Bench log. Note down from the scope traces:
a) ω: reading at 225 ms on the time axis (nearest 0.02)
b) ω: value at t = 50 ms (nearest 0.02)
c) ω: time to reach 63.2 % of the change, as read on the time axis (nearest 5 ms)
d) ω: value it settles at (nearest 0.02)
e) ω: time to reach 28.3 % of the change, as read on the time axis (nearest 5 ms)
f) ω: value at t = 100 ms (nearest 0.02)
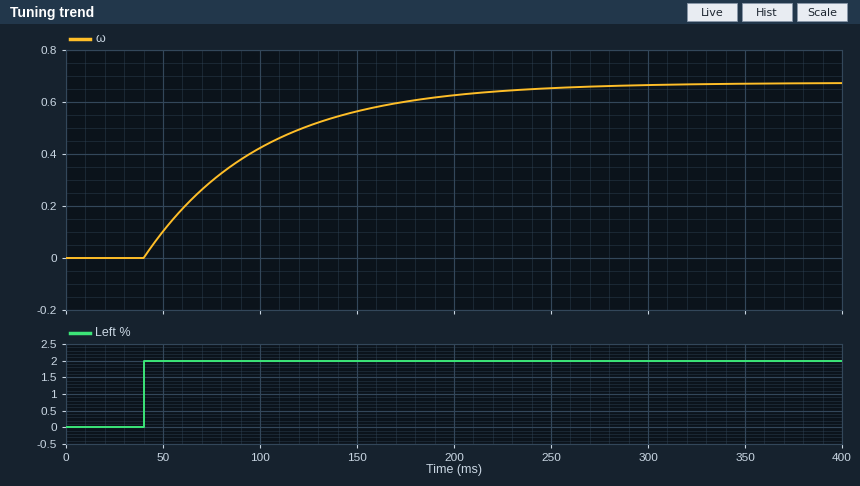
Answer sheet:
0.64
0.10
100 ms
0.68
60 ms
0.42
